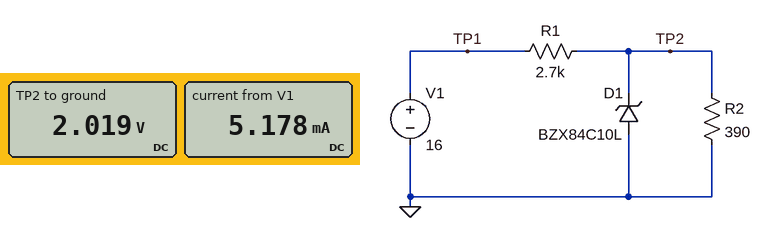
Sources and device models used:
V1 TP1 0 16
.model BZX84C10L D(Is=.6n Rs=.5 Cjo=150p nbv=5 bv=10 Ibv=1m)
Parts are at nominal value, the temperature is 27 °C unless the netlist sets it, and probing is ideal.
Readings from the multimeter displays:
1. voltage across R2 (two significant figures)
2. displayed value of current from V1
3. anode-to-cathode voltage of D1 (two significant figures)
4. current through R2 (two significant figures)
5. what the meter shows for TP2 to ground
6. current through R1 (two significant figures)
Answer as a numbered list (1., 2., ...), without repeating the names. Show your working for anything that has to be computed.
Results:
1. 2.019 V = 2.0 V
2. 5.178 mA
3. 0 V - 2.019 V = -2.0 V
4. (2.019 V) / 390 Ω = 5.2 mA
5. 2.019 V
6. (16 V - 2.019 V) / 2.7 kΩ = 5.2 mA
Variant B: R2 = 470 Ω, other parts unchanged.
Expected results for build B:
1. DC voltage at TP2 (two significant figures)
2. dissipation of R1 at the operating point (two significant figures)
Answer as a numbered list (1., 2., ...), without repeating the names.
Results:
1. 2.4 V
2. 69 mW
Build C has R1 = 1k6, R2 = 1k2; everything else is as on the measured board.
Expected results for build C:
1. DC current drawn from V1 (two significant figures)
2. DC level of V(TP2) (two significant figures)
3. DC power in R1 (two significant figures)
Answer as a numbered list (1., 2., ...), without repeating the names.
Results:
1. 5.7 mA
2. 6.9 V
3. 52 mW
